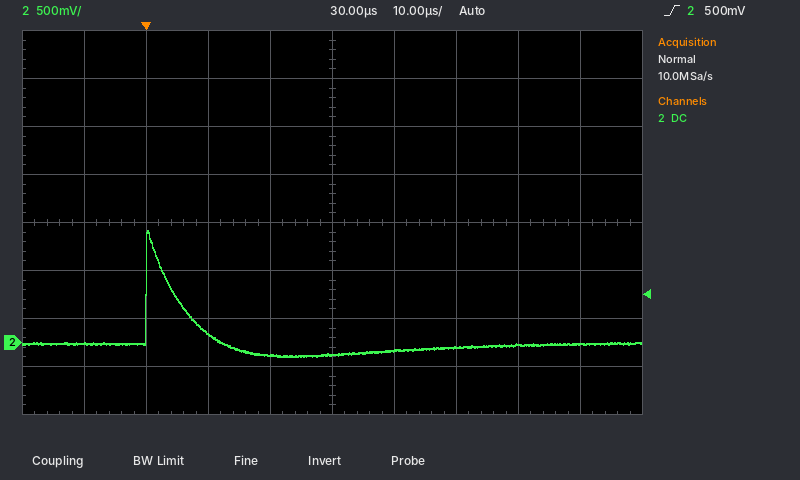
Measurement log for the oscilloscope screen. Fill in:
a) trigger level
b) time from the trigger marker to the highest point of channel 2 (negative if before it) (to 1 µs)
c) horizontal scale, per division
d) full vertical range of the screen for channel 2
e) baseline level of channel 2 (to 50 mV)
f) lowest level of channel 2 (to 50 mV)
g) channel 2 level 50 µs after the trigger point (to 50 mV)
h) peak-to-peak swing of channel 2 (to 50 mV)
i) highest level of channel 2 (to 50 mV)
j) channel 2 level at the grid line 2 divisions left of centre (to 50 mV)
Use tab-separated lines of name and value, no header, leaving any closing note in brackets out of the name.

trigger level	500 mV
time from the trigger marker to the highest point of channel 2 (negative if before it)	0 µs
horizontal scale, per division	10 µs
full vertical range of the screen for channel 2	4 V
baseline level of channel 2	0 mV
lowest level of channel 2	-150 mV
channel 2 level 50 µs after the trigger point	-50 mV
peak-to-peak swing of channel 2	1.30 V
highest level of channel 2	1.15 V
channel 2 level at the grid line 2 divisions left of centre	100 mV
